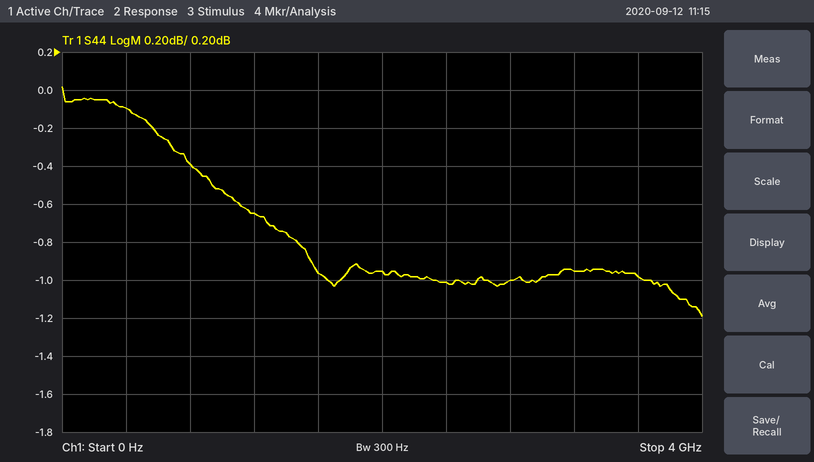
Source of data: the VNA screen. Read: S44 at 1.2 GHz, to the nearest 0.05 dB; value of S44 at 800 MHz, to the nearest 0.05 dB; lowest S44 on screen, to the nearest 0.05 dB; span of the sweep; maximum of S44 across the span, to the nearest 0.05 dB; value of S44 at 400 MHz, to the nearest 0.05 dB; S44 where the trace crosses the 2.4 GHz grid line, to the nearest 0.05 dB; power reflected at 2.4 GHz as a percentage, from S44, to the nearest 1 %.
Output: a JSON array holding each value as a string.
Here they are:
["-0.65 dB", "-0.40 dB", "-1.20 dB", "4 GHz", "0.00 dB", "-0.10 dB", "-1.00 dB", "79 %"]
